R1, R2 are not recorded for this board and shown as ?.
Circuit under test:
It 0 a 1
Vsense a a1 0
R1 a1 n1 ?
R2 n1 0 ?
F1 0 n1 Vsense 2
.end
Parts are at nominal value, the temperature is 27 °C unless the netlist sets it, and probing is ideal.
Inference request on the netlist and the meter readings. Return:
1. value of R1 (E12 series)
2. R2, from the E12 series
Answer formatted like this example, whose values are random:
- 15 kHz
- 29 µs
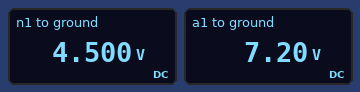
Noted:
- 2.7 Ω
- 1.5 Ω
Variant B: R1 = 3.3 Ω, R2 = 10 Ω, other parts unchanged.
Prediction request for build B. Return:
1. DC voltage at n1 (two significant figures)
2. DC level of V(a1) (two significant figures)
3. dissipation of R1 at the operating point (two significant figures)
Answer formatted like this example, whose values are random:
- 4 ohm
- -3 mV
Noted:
- 30 V
- 33 V
- 3.3 W
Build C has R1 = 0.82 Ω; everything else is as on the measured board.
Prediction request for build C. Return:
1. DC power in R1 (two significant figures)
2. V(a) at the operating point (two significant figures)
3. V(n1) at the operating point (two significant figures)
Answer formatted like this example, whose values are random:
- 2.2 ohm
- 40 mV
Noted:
- 820 mW
- 5.3 V
- 4.5 V
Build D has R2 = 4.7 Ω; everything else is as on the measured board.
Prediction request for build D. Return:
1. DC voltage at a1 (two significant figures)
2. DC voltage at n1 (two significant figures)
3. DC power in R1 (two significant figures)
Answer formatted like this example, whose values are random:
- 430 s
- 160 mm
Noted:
- 17 V
- 14 V
- 2.7 W
